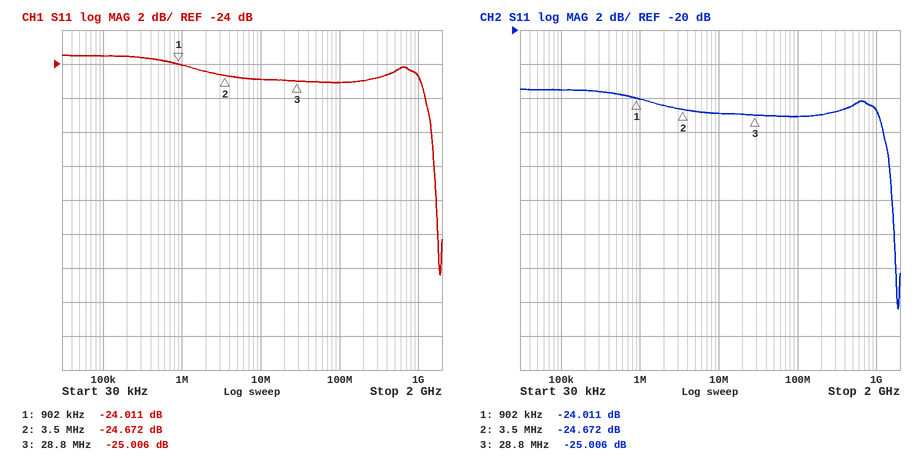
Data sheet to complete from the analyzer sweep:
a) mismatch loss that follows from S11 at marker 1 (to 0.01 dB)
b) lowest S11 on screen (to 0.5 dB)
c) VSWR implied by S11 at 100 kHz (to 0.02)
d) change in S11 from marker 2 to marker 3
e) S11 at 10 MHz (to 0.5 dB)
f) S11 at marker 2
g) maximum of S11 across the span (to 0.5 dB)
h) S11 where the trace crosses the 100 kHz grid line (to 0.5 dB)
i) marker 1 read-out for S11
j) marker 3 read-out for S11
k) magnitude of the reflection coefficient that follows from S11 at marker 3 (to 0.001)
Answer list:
0.02 dB
-36.5 dB
1.14
-0.334 dB
-25.0 dB
-24.672 dB
-23.5 dB
-23.5 dB
-24.011 dB
-25.006 dB
0.056
